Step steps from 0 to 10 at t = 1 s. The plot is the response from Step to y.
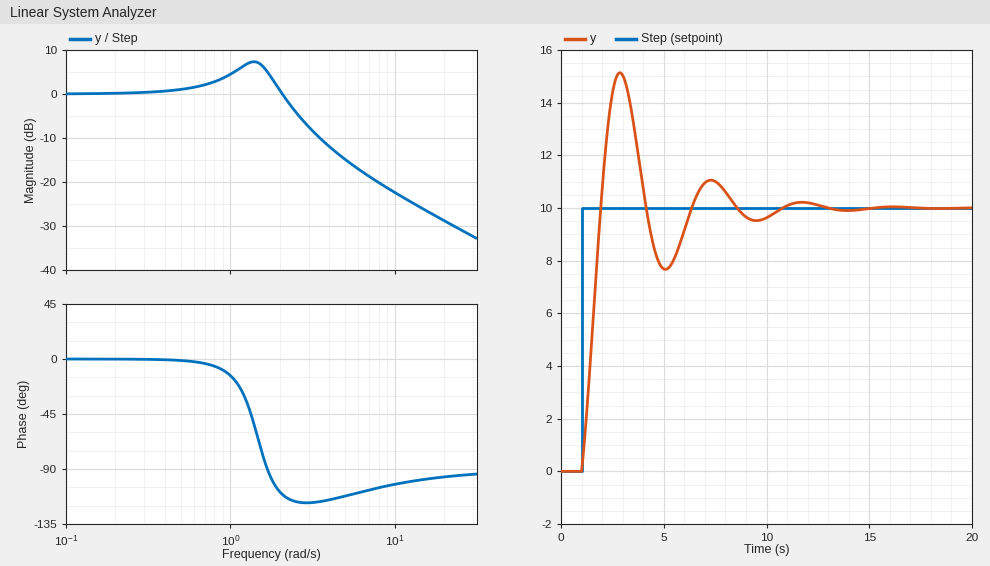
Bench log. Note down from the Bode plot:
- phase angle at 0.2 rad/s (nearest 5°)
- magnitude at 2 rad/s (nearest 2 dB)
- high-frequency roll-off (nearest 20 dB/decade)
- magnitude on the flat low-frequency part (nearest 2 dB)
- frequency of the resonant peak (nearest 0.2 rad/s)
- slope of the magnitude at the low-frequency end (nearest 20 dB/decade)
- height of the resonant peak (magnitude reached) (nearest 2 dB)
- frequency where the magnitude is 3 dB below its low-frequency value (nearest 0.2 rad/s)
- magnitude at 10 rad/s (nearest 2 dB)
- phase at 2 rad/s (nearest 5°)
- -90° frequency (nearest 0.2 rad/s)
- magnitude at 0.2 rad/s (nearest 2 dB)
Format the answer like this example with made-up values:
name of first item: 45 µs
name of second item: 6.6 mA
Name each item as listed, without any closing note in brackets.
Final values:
phase angle at 0.2 rad/s: 0°
magnitude at 2 rad/s: 0 dB
high-frequency roll-off: -20 dB/decade
magnitude on the flat low-frequency part: 0 dB
frequency of the resonant peak: 1.4 rad/s
slope of the magnitude at the low-frequency end: 0 dB/decade
height of the resonant peak (magnitude reached): 8 dB
frequency where the magnitude is 3 dB below its low-frequency value: 2.4 rad/s
magnitude at 10 rad/s: -22 dB
phase at 2 rad/s: -110°
-90° frequency: 1.6 rad/s
magnitude at 0.2 rad/s: 0 dB
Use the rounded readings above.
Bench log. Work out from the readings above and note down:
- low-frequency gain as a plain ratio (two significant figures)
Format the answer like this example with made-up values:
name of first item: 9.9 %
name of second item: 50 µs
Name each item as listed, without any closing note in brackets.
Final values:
low-frequency gain as a plain ratio: 1.0
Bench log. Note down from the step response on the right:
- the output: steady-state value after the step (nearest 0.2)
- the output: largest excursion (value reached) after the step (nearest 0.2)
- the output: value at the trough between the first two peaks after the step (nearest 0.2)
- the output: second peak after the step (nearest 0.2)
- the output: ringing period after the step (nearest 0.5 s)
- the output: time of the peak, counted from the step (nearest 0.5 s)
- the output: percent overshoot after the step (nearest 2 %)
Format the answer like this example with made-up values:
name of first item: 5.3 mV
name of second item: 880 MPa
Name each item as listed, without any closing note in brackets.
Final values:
the output: steady-state value after the step: 10.0
the output: largest excursion (value reached) after the step: 15.2
the output: value at the trough between the first two peaks after the step: 7.6
the output: second peak after the step: 11.0
the output: ringing period after the step: 4.5 s
the output: time of the peak, counted from the step: 2.0 s
the output: percent overshoot after the step: 52 %
